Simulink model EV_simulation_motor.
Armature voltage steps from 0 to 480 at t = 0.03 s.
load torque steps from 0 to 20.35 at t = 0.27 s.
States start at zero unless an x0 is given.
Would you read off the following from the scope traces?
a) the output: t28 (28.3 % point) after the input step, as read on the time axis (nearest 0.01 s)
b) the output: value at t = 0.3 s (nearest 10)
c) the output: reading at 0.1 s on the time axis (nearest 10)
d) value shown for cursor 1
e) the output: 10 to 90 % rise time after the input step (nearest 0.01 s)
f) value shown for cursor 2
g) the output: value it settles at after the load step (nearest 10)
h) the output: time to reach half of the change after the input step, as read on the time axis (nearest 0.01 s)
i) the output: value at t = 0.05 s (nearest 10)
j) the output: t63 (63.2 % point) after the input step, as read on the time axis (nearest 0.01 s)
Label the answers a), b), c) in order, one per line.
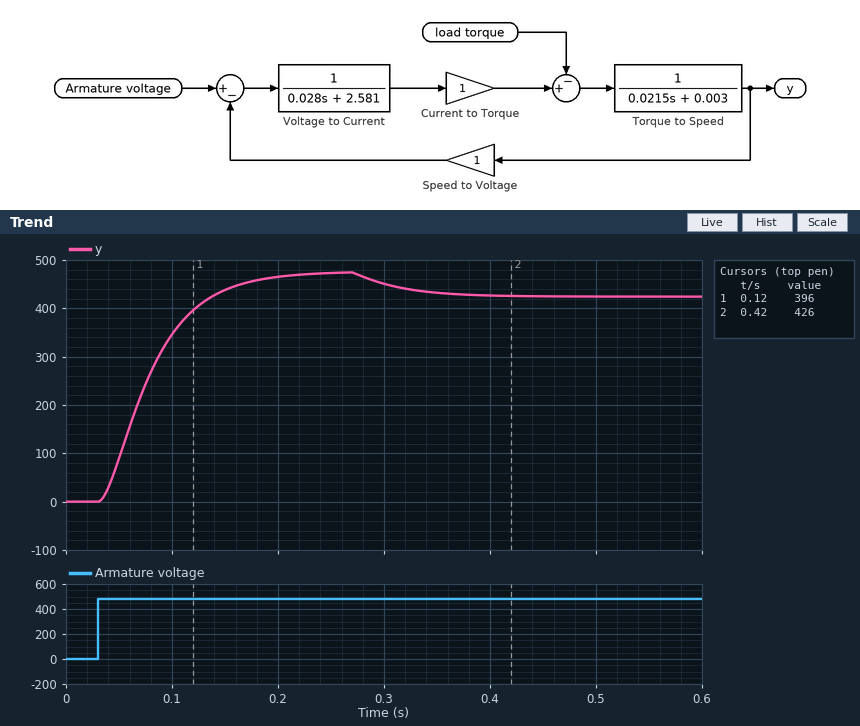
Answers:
a) 0.06 s
b) 450
c) 350
d) 396
e) 0.10 s
f) 426
g) 420
h) 0.07 s
i) 90
j) 0.09 s
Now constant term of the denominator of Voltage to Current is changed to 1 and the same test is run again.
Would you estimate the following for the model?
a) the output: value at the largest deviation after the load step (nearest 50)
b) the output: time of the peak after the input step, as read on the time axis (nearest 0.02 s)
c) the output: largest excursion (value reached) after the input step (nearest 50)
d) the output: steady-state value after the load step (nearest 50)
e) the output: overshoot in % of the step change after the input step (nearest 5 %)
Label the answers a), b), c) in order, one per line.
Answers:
a) 450
b) 0.12 s
c) 600
d) 450
e) 20 %
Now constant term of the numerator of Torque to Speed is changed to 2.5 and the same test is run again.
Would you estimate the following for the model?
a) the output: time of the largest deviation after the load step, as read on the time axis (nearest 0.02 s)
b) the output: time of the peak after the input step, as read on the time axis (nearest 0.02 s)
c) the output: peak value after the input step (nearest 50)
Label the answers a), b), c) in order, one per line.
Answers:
a) 0.32 s
b) 0.10 s
c) 500
